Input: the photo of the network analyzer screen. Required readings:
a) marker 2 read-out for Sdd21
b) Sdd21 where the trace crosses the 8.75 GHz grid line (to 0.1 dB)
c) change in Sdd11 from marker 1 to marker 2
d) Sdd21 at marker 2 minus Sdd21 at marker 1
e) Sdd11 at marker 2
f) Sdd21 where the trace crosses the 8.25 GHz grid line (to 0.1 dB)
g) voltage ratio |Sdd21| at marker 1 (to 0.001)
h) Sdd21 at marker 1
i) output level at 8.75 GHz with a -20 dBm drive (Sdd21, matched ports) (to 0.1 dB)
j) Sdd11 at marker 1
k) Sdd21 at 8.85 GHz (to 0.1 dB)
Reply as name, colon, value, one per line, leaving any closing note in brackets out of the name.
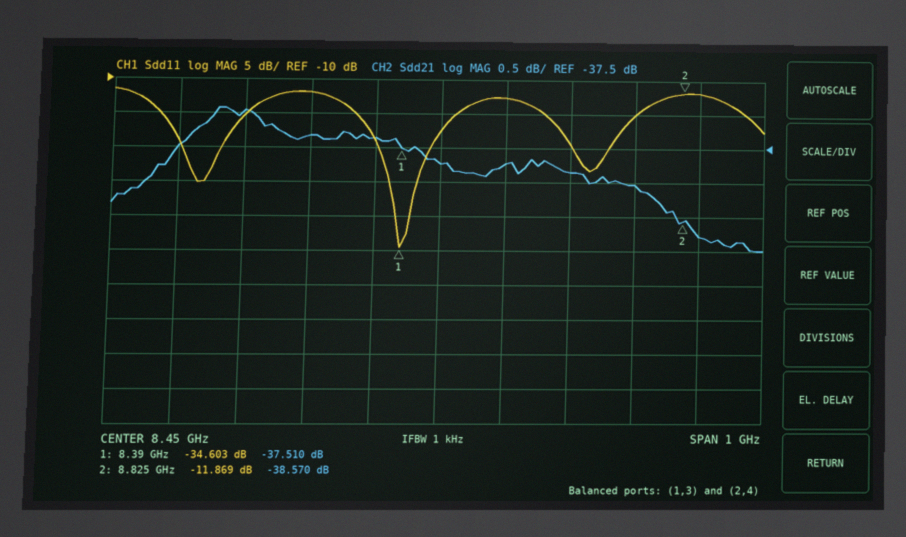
marker 2 read-out for Sdd21: -38.570 dB
Sdd21 where the trace crosses the 8.75 GHz grid line: -38.0 dB
change in Sdd11 from marker 1 to marker 2: 22.734 dB
Sdd21 at marker 2 minus Sdd21 at marker 1: -1.060 dB
Sdd11 at marker 2: -11.869 dB
Sdd21 where the trace crosses the 8.25 GHz grid line: -37.3 dB
voltage ratio |Sdd21| at marker 1: 0.013
Sdd21 at marker 1: -37.510 dB
output level at 8.75 GHz with a -20 dBm drive (Sdd21, matched ports): -58.0 dBm
Sdd11 at marker 1: -34.603 dB
Sdd21 at 8.85 GHz: -38.8 dB
